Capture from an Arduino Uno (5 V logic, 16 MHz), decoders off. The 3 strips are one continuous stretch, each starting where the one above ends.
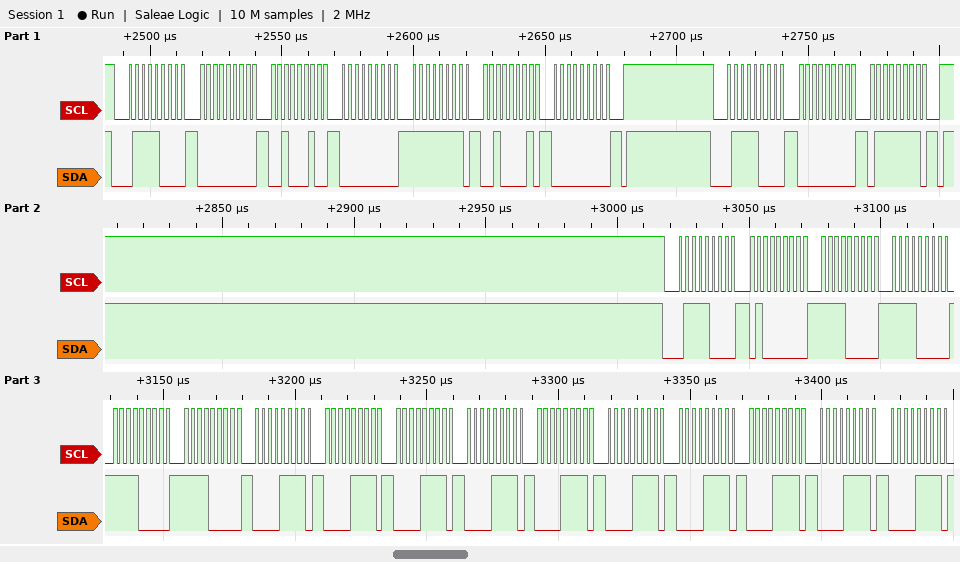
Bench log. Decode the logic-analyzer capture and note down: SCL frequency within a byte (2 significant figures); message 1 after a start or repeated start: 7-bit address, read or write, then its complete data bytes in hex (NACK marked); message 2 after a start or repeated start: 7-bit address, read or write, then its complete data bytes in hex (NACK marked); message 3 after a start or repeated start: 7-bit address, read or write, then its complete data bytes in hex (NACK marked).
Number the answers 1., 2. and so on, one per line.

1. 400 kHz
2. 0x3C write: 00 22 00 FF 21 00
3. 0x3C write: 00 7F
4. 0x3C write: 40 F0 F0 F0 F0 0F 0F 0F 0F 0F 0F 0F 0F 0F 0F
